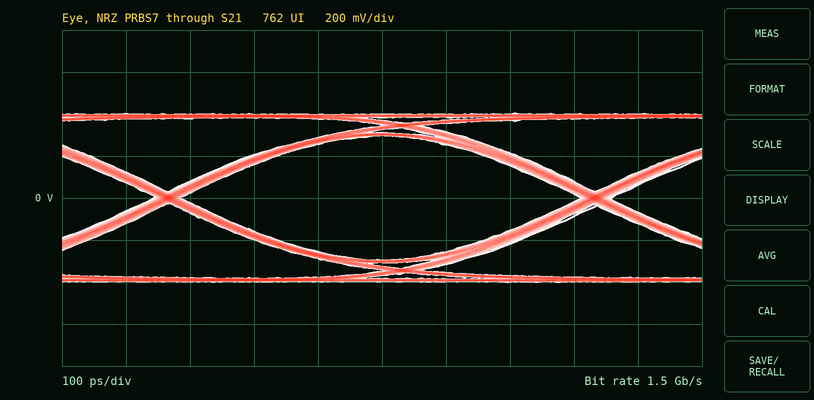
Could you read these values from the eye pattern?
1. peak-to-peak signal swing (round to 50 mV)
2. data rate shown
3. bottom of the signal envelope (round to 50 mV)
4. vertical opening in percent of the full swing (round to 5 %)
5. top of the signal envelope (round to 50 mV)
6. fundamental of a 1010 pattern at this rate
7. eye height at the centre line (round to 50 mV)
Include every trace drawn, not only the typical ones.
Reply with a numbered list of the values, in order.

1. 800 mV
2. 1.5 Gb/s
3. -400 mV
4. 75 %
5. 400 mV
6. 750 MHz
7. 600 mV
